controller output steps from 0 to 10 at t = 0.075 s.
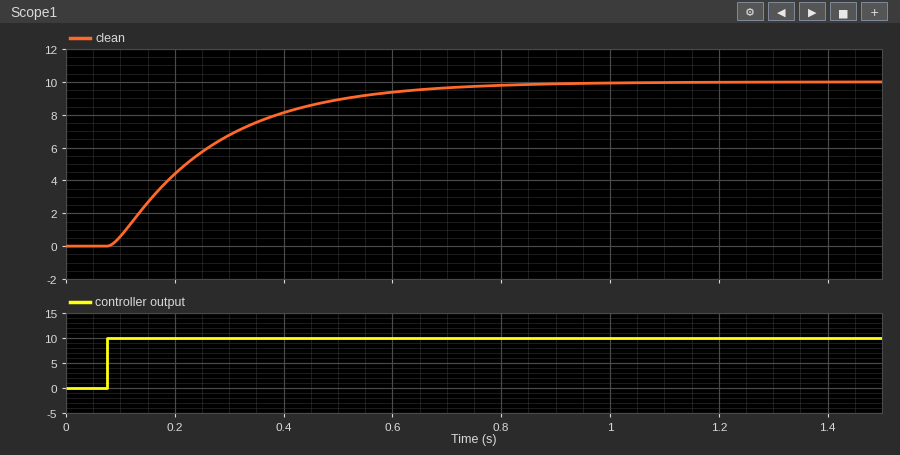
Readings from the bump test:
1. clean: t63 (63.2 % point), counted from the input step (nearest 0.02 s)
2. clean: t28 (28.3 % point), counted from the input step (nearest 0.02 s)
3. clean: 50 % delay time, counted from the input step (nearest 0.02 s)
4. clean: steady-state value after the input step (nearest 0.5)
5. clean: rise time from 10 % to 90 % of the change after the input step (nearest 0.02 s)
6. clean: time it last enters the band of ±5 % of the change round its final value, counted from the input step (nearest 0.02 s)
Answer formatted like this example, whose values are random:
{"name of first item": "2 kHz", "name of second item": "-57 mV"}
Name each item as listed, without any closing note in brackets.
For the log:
{"clean: t63 (63.2 % point), counted from the input step": "0.20 s", "clean: t28 (28.3 % point), counted from the input step": "0.08 s", "clean: 50 % delay time, counted from the input step": "0.14 s", "clean: steady-state value after the input step": "10.0", "clean: rise time from 10 % to 90 % of the change after the input step": "0.40 s", "clean: time it last enters the band of ±5 % of the change round its final value, counted from the input step": "0.56 s"}
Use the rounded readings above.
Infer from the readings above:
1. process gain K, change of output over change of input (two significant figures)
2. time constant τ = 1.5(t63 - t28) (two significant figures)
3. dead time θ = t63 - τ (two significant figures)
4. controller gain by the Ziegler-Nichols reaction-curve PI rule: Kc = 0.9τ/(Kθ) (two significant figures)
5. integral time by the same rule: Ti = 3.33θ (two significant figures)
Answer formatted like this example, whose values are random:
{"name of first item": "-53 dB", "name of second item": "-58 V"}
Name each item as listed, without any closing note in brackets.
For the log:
{"process gain K, change of output over change of input": "1.0", "time constant τ = 1.5(t63 - t28)": "0.18 s", "dead time θ = t63 - τ": "0.020 s", "controller gain by the Ziegler-Nichols reaction-curve PI rule: Kc = 0.9τ/(Kθ)": "8.1", "integral time by the same rule: Ti = 3.33θ": "0.067 s"}
